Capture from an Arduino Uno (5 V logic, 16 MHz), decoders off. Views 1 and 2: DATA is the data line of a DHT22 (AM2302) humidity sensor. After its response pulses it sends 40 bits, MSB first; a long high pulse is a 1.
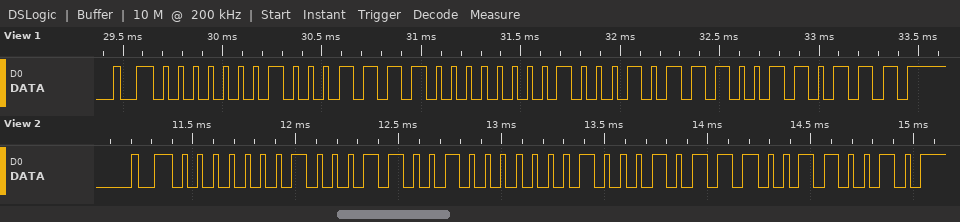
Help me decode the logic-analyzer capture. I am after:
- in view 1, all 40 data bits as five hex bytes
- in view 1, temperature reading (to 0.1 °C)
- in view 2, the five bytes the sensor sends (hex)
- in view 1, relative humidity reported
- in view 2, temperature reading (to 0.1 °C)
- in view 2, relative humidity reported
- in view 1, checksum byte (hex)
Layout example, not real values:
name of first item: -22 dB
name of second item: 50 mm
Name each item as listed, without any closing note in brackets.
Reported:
in view 1, all 40 data bits as five hex bytes: 01 1E 01 17 37
in view 1, temperature reading: 27.9 °C
in view 2, the five bytes the sensor sends: 01 19 01 17 32
in view 1, relative humidity reported: 28.6 %
in view 2, temperature reading: 27.9 °C
in view 2, relative humidity reported: 28.1 %
in view 1, checksum byte: 0x37
